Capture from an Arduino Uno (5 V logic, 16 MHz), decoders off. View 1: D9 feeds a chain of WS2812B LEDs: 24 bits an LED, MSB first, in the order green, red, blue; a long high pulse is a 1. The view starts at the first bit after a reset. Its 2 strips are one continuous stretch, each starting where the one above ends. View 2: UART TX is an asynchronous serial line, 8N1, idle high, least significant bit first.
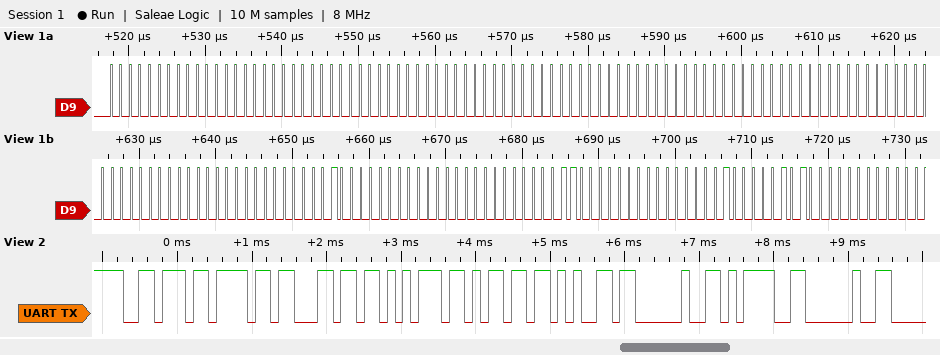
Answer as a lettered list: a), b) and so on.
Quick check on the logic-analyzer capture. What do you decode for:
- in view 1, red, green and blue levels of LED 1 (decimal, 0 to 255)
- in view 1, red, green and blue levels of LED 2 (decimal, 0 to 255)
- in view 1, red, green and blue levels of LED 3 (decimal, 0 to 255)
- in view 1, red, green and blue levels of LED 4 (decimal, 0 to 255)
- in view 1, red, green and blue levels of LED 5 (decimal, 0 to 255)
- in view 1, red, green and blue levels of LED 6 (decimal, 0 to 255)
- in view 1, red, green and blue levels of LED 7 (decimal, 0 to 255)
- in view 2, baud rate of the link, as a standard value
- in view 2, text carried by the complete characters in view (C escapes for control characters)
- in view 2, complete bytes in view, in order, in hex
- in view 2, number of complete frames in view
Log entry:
a) 0, 0, 0
b) 0, 0, 0
c) 0, 0, 0
d) 0, 0, 0
e) 2, 0, 0
f) 3, 0, 0
g) 5, 1, 0
h) 9600 baud
i) "volume = "
j) 76 6F 6C 75 6D 65 20 3D 20
k) 9
